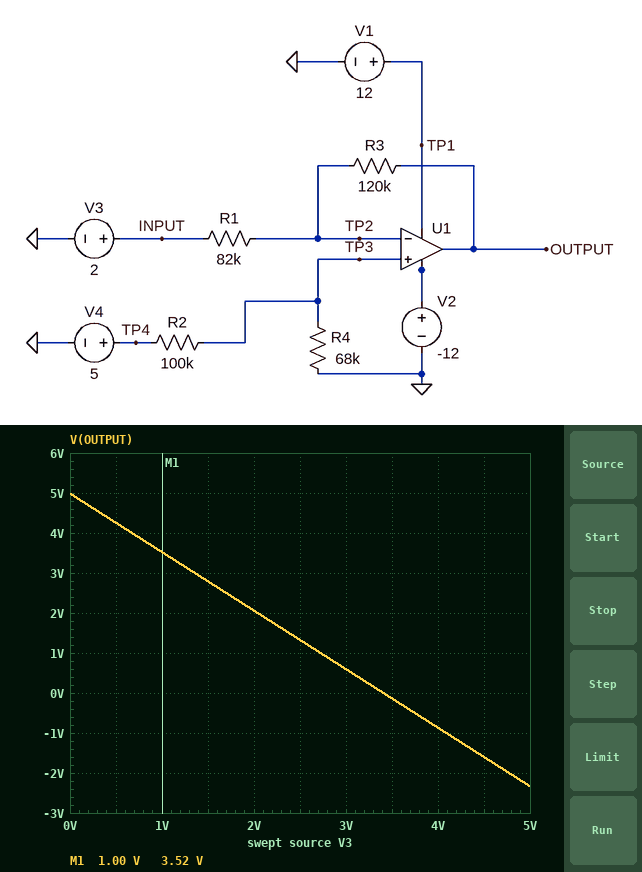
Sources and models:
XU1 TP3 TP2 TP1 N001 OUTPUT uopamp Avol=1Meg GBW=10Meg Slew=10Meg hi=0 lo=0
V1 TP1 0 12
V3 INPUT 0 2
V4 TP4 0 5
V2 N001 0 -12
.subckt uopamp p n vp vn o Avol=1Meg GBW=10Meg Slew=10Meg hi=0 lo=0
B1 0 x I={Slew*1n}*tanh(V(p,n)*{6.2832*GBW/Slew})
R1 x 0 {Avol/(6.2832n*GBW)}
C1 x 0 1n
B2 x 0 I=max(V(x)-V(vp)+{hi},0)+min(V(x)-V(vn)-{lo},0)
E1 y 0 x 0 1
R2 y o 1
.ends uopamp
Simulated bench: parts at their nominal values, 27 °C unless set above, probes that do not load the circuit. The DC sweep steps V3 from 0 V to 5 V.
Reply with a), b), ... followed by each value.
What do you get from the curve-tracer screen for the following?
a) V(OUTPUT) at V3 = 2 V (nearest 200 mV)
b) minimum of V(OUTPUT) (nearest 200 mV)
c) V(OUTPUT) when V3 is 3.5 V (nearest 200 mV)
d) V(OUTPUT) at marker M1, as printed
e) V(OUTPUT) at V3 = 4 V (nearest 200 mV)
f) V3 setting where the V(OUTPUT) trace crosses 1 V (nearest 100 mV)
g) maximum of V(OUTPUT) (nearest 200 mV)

a) 2.0 V
b) -2.4 V
c) -200 mV
d) 3.52 V
e) -800 mV
f) 2.7 V
g) 5.0 V
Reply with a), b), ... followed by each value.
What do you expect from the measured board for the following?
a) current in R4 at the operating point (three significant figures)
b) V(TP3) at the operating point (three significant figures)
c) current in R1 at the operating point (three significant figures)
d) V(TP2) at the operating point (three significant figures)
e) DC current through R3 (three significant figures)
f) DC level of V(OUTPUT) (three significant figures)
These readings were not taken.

a) 29.8 µA
b) 2.02 V
c) 290 nA
d) 2.02 V
e) 290 nA
f) 2.06 V
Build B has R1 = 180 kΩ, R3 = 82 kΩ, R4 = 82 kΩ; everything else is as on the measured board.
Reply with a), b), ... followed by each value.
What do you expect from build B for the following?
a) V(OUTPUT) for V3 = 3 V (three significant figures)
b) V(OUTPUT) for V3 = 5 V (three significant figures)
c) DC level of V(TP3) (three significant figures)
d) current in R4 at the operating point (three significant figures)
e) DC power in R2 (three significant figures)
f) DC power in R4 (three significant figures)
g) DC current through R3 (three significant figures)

a) 1.91 V
b) 1.00 V
c) 2.25 V
d) 27.5 µA
e) 75.5 µW
f) 61.9 µW
g) 1.40 µA
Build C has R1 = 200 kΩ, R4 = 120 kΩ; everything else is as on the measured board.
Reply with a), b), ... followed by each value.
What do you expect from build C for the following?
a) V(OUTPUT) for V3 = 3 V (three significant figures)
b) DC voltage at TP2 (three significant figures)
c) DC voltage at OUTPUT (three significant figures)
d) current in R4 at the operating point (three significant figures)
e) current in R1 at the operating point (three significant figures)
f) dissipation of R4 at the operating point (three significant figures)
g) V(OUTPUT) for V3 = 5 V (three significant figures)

a) 2.56 V
b) 2.73 V
c) 3.16 V
d) 22.7 µA
e) 3.64 µA
f) 62.0 µW
g) 1.36 V
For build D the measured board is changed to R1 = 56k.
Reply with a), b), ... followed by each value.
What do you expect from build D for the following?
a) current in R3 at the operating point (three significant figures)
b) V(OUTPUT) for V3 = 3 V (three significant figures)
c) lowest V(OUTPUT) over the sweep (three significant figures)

a) 425 nA
b) -68.0 mV
c) -4.35 V
